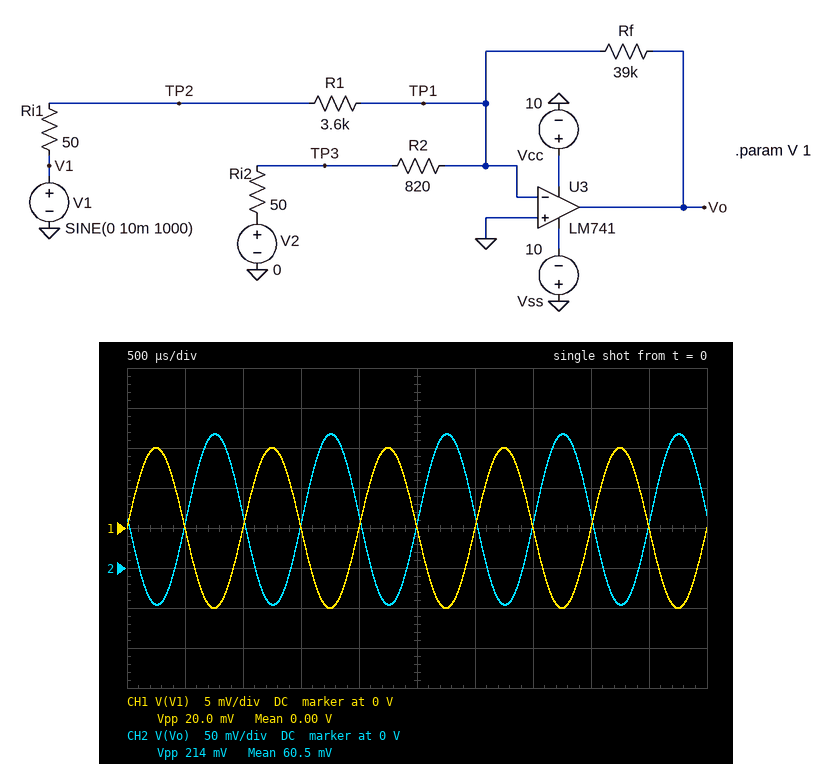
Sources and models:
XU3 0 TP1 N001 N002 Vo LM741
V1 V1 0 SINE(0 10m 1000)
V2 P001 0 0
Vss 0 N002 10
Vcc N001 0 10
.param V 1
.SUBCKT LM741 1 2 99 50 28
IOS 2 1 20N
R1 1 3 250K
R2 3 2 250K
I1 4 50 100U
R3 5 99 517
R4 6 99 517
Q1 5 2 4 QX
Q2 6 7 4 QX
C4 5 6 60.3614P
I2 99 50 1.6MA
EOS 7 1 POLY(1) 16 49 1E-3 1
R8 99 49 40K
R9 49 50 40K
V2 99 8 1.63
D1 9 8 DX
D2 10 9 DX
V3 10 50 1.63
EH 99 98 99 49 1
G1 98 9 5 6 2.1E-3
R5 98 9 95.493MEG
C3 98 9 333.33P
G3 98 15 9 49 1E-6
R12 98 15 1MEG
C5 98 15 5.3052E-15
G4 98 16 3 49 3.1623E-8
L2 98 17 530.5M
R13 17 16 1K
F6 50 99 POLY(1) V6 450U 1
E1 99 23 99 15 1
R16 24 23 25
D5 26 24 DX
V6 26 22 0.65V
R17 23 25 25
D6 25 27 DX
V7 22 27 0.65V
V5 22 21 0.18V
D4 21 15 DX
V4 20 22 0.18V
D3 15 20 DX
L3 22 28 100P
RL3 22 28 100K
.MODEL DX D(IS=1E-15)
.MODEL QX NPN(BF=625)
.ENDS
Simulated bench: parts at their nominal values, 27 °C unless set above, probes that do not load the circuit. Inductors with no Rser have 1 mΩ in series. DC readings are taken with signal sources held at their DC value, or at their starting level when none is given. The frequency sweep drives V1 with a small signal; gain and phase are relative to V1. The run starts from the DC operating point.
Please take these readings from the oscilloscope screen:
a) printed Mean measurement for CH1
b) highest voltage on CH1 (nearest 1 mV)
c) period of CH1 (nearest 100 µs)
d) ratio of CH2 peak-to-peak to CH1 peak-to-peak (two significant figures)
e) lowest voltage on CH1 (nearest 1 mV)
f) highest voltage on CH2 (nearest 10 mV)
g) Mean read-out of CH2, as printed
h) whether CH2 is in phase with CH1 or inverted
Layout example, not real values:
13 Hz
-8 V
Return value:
0.00 V
10 mV
1.0 ms
11
-10 mV
170 mV
60.5 mV
inverted
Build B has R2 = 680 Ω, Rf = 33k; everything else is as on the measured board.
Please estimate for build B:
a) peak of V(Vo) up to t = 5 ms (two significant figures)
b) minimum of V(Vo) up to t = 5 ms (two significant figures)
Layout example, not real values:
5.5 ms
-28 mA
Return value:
150 mV
-32 mV
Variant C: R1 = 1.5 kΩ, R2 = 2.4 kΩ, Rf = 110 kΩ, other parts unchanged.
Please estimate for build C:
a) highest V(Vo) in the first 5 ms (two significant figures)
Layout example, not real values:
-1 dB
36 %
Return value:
830 mV
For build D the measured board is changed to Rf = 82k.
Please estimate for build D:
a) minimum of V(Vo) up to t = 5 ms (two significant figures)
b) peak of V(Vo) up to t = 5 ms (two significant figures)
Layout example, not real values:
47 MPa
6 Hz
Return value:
-97 mV
350 mV
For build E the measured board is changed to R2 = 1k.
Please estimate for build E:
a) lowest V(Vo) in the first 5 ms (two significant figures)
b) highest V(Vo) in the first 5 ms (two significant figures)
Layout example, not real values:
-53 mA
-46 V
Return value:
-54 mV
160 mV
